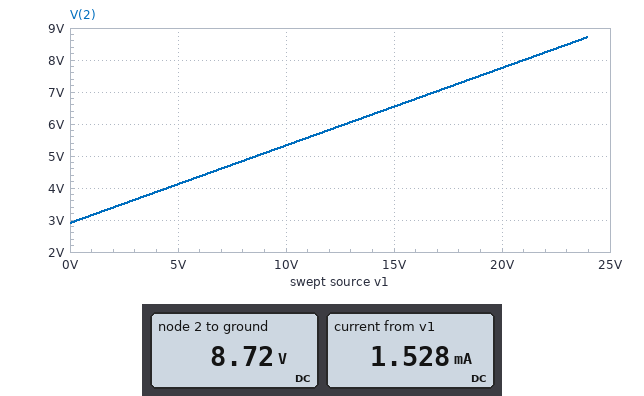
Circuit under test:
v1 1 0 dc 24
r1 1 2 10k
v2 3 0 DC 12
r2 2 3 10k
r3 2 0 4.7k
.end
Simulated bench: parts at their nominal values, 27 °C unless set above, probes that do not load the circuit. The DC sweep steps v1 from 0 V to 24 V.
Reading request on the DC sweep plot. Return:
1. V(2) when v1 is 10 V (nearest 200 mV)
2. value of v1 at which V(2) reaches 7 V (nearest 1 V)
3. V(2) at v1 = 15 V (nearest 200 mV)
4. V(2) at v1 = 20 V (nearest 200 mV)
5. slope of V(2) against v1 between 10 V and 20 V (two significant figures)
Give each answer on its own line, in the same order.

5.4 V
17 V
6.6 V
7.8 V
0.24 V/V
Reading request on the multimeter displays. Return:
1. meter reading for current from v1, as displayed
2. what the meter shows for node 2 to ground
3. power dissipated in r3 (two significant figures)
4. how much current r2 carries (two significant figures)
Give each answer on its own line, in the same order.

1.528 mA
8.72 V
16 mW
330 µA
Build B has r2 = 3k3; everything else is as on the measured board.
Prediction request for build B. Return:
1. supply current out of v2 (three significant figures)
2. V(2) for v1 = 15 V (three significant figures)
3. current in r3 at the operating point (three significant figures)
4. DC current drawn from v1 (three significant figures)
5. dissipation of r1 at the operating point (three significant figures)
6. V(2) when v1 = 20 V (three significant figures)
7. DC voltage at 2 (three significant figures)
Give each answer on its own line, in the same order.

666 µA
8.34 V
2.09 mA
1.42 mA
20.2 mW
9.15 V
9.80 V
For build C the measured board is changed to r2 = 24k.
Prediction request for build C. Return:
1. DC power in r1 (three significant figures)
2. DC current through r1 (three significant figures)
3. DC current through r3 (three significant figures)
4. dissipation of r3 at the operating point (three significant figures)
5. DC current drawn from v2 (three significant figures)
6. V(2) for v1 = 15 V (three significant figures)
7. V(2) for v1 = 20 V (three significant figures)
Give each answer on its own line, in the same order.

25.0 mW
1.58 mA
1.74 mA
14.2 mW
159 µA
5.64 V
7.05 V
